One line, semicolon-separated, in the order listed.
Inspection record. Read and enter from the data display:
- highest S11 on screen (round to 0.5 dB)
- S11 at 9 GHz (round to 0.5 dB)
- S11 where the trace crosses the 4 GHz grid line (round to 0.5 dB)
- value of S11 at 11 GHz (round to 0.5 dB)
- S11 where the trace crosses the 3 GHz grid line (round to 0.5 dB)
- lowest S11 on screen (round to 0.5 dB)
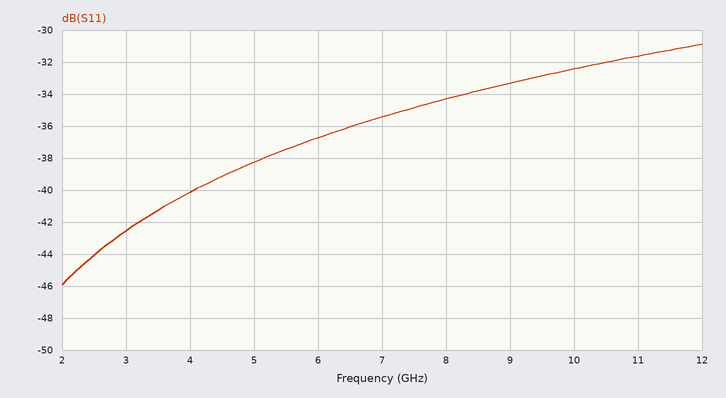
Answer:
-31.0 dB; -33.5 dB; -40.0 dB; -31.5 dB; -42.5 dB; -46.0 dB
